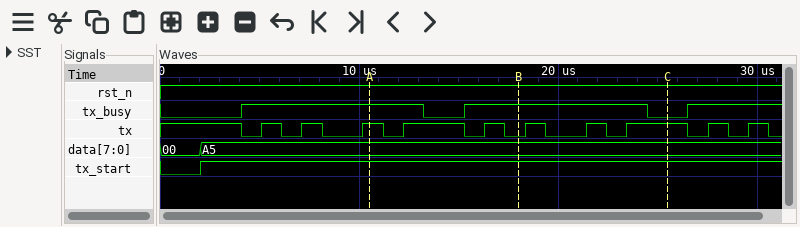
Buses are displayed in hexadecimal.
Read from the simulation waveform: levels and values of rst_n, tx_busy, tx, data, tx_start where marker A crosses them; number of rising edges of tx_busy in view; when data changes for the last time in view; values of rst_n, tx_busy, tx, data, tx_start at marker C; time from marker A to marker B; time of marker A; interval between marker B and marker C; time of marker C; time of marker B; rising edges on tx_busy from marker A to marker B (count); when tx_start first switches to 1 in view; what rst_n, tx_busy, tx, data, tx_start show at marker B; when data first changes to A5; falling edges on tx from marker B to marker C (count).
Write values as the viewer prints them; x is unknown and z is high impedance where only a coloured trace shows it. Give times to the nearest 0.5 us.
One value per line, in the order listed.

rst_n=1, tx_busy=1, tx=1, data=A5, tx_start=1
3
2 us
rst_n=1, tx_busy=0, tx=1, data=A5, tx_start=1
7.5 us
10.5 us
7.5 us
25.5 us
18 us
1
2 us
rst_n=1, tx_busy=1, tx=0, data=A5, tx_start=1
2 us
2
